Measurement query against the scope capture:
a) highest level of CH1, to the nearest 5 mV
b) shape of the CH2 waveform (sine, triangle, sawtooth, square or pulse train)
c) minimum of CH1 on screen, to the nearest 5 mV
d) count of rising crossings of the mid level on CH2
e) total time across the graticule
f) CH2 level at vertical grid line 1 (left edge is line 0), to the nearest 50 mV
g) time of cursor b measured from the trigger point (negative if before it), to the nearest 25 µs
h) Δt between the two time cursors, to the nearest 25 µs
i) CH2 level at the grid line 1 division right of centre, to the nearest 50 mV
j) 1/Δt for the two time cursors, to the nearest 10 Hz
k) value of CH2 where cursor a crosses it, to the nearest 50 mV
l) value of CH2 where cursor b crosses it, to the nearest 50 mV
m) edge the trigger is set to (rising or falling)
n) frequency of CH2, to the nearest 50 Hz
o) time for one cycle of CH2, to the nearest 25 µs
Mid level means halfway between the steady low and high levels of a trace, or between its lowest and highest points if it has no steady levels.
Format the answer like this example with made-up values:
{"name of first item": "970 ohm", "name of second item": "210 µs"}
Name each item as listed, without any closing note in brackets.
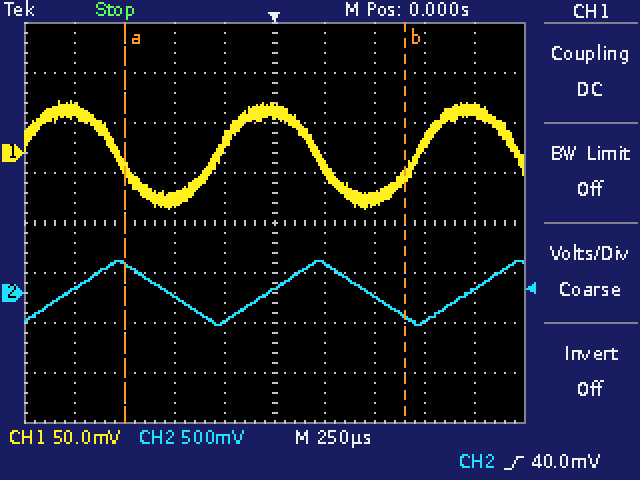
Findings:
{"highest level of CH1, to the nearest 5 mV": "50 mV", "shape of the CH2 waveform": "triangle", "minimum of CH1 on screen, to the nearest 5 mV": "-55 mV", "count of rising crossings of the mid level on CH2": "3", "total time across the graticule": "2.5 ms", "CH2 level at vertical grid line 1 (left edge is line 0), to the nearest 50 mV": "50 mV", "time of cursor b measured from the trigger point (negative if before it), to the nearest 25 µs": "+650 µs", "Δt between the two time cursors, to the nearest 25 µs": "1.400 ms", "CH2 level at the grid line 1 division right of centre, to the nearest 50 mV": "300 mV", "1/Δt for the two time cursors, to the nearest 10 Hz": "710 Hz", "value of CH2 where cursor a crosses it, to the nearest 50 mV": "300 mV", "value of CH2 where cursor b crosses it, to the nearest 50 mV": "-250 mV", "edge the trigger is set to": "rising", "frequency of CH2, to the nearest 50 Hz": "1.00 kHz", "time for one cycle of CH2, to the nearest 25 µs": "1.000 ms"}
